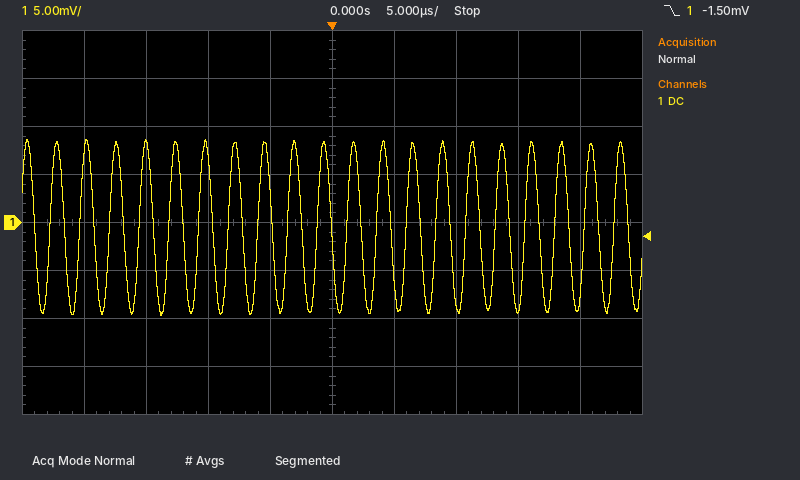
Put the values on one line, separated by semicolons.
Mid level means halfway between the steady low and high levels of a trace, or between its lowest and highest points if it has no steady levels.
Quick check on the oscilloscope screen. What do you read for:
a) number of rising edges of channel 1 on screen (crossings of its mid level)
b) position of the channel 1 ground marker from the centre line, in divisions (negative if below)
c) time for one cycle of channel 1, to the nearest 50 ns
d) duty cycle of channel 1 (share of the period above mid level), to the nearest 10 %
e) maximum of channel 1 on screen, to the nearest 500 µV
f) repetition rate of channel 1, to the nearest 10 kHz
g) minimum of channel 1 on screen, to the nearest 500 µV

20; 0.0 div; 2.40 µs; 50 %; 8.5 mV; 420 kHz; -9.5 mV
